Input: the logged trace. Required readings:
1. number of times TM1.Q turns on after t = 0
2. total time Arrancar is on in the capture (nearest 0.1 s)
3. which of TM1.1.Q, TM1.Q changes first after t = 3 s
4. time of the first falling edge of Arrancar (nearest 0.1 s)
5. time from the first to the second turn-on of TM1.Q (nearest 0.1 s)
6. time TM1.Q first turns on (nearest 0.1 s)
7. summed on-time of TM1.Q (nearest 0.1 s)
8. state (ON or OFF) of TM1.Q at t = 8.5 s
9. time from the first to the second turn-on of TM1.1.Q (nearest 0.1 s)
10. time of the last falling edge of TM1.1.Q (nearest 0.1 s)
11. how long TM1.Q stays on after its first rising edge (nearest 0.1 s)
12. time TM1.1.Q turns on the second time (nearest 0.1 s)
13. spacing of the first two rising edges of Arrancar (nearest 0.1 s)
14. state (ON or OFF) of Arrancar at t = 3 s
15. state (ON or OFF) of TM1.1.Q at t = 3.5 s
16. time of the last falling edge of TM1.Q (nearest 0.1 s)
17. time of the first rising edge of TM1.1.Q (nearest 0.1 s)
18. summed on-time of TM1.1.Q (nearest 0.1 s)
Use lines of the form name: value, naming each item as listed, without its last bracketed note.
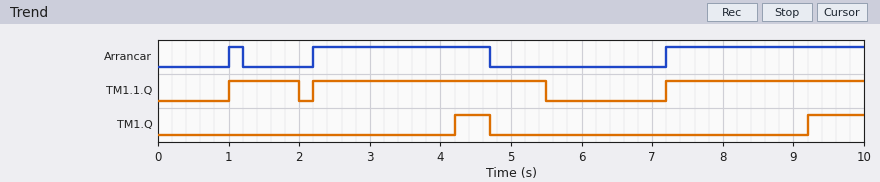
number of times TM1.Q turns on after t = 0: 2
total time Arrancar is on in the capture: 5.5 s
which of TM1.1.Q, TM1.Q changes first after t = 3 s: TM1.Q
time of the first falling edge of Arrancar: 1.2 s
time from the first to the second turn-on of TM1.Q: 5.0 s
time TM1.Q first turns on: 4.2 s
summed on-time of TM1.Q: 1.3 s
state (ON or OFF) of TM1.Q at t = 8.5 s: OFF
time from the first to the second turn-on of TM1.1.Q: 1.2 s
time of the last falling edge of TM1.1.Q: 5.5 s
how long TM1.Q stays on after its first rising edge: 0.5 s
time TM1.1.Q turns on the second time: 2.2 s
spacing of the first two rising edges of Arrancar: 1.2 s
state (ON or OFF) of Arrancar at t = 3 s: ON
state (ON or OFF) of TM1.1.Q at t = 3.5 s: ON
time of the last falling edge of TM1.Q: 4.7 s
time of the first rising edge of TM1.1.Q: 1.0 s
summed on-time of TM1.1.Q: 7.1 s
